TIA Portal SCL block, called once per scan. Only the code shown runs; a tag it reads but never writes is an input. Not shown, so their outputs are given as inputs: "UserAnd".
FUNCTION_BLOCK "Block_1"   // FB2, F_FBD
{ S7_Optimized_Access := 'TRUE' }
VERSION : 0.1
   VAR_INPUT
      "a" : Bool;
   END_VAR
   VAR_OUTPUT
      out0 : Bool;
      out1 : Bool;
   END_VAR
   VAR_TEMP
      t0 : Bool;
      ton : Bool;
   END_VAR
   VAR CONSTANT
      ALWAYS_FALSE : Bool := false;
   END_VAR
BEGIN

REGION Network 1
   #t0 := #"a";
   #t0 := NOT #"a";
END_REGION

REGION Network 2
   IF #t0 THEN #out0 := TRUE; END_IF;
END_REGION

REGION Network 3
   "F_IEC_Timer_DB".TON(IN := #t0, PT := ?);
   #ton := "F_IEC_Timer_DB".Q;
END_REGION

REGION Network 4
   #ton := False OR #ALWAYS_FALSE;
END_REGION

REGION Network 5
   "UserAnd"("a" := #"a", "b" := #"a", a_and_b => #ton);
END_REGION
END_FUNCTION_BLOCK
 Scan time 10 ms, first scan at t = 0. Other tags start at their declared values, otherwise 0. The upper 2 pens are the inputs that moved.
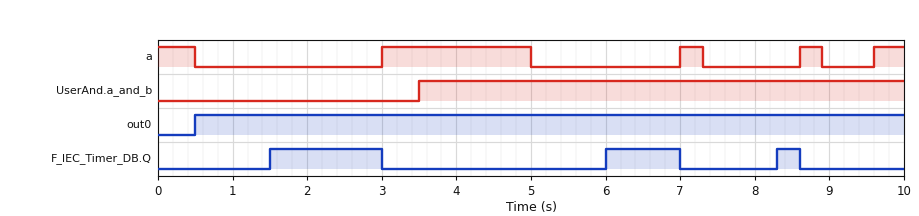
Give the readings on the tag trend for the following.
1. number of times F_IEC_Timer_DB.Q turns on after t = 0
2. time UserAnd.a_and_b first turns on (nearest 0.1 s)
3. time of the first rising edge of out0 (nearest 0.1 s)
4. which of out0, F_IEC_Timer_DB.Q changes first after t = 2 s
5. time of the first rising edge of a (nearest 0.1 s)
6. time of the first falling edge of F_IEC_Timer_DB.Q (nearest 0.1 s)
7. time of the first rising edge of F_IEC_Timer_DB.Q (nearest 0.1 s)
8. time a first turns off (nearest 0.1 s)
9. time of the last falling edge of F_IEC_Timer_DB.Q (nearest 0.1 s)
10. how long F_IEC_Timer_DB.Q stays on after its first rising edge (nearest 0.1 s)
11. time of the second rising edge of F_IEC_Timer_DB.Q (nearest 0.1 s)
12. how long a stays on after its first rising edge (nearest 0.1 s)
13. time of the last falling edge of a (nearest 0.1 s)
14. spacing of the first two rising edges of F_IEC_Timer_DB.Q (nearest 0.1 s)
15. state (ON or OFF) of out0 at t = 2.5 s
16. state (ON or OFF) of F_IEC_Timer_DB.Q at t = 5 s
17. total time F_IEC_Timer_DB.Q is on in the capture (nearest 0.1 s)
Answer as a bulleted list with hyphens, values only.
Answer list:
- 3
- 3.5 s
- 0.5 s
- F_IEC_Timer_DB.Q
- 3.0 s
- 3.0 s
- 1.5 s
- 0.5 s
- 8.6 s
- 1.5 s
- 6.0 s
- 2.0 s
- 8.9 s
- 4.5 s
- ON
- OFF
- 2.8 s
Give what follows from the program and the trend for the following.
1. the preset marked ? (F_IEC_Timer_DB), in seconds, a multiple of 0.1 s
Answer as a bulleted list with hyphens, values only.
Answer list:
- 1.0 s
